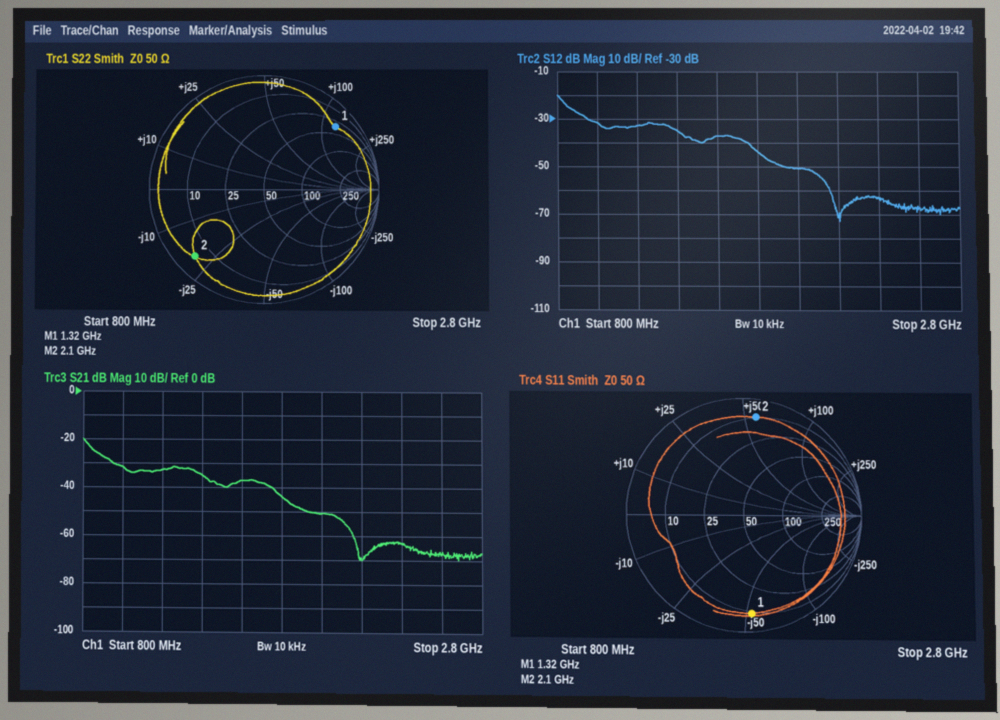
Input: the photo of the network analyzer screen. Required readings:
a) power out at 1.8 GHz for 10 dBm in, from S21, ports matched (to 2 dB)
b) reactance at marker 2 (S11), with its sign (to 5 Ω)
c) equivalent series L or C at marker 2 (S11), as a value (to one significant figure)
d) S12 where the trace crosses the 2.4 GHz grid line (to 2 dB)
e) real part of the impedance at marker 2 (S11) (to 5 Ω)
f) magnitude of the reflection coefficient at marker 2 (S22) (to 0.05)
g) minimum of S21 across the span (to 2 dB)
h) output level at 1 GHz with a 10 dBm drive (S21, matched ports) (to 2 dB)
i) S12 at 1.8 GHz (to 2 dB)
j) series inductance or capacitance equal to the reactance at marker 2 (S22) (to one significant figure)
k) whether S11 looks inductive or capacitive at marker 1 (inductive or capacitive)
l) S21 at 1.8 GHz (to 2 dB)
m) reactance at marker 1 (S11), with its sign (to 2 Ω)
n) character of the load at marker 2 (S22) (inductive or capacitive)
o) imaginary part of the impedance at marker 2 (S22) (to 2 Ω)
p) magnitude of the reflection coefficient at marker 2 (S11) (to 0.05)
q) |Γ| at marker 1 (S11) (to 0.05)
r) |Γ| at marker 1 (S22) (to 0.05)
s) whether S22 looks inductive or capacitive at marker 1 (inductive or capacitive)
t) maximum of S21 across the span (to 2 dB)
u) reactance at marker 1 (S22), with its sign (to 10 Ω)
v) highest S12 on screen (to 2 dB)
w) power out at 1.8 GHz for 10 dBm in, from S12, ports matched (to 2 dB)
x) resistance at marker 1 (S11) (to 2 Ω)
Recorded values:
-34 dBm
+55 Ω
4 nH
-64 dB
10 Ω
0.85
-70 dB
-22 dBm
-44 dB
4 pF
capacitive
-44 dB
-52 Ω
capacitive
-20 Ω
0.85
0.85
0.85
inductive
-20 dB
+120 Ω
-20 dB
-34 dBm
10 Ω
